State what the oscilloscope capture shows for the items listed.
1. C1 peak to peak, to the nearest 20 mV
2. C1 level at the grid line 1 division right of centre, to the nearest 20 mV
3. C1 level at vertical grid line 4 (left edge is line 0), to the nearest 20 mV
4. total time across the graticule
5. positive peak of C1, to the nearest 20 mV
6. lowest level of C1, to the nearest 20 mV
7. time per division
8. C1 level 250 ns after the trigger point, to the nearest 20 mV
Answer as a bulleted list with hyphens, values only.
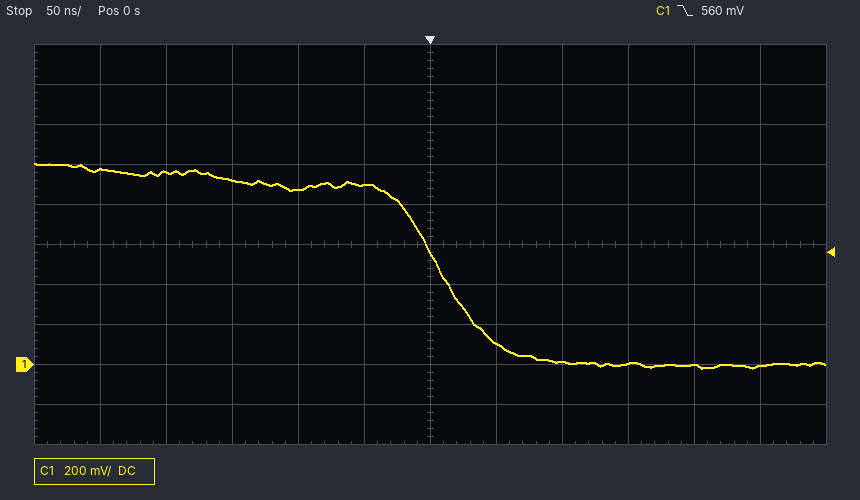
- 1.02 V
- 100 mV
- 880 mV
- 600 ns
- 1.00 V
- -20 mV
- 50 ns
- 0 mV
